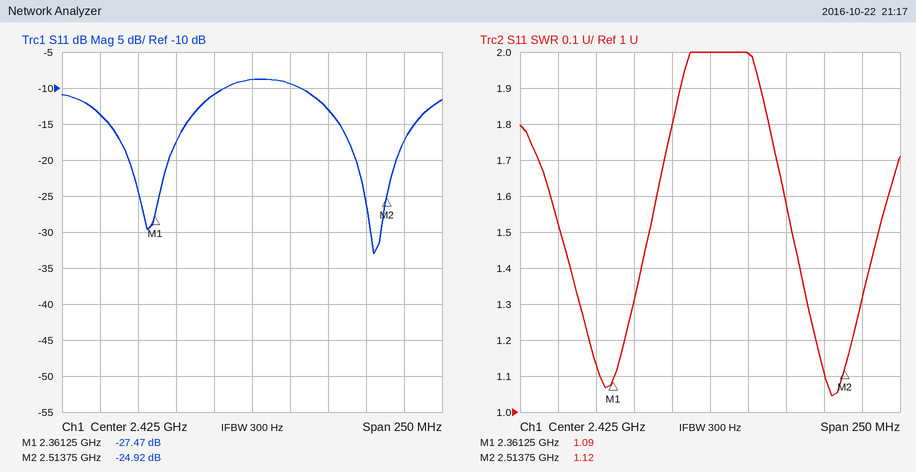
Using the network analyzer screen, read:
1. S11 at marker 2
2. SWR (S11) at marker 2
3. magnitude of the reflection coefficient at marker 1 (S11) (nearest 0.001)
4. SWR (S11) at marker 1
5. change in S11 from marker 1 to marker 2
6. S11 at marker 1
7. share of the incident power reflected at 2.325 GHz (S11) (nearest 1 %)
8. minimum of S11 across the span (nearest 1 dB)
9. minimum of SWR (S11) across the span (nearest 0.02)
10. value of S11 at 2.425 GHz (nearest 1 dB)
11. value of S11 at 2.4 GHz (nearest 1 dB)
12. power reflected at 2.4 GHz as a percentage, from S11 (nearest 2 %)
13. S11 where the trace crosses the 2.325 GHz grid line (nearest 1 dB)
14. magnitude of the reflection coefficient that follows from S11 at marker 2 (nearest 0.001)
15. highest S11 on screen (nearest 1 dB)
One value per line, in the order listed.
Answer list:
-24.92 dB
1.12
0.042
1.09
2.55 dB
-27.47 dB
4 %
-33 dB
1.04
-9 dB
-11 dB
8 %
-14 dB
0.057
-9 dB
